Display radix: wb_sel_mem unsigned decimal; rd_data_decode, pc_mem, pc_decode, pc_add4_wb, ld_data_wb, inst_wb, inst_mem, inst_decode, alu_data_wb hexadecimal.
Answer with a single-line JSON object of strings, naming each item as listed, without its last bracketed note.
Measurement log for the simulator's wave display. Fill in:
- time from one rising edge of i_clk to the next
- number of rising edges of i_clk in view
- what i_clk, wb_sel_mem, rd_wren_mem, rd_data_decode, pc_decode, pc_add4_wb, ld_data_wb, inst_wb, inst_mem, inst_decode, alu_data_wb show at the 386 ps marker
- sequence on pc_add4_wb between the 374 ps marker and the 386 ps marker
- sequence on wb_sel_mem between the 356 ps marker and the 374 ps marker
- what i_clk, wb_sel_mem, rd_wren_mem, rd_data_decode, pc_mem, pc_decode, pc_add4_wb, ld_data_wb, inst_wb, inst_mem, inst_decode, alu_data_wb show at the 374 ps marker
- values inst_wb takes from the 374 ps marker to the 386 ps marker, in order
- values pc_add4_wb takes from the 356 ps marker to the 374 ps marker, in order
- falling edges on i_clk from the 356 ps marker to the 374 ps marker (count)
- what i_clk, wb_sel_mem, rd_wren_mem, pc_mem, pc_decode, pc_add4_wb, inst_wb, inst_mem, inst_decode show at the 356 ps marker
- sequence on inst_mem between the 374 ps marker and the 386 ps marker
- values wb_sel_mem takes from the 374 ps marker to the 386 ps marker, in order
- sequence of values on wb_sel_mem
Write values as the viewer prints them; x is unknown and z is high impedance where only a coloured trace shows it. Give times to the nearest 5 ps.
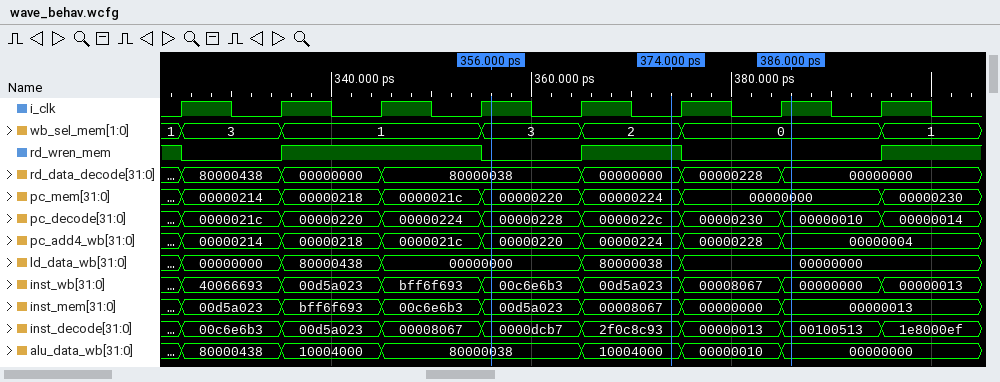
{"time from one rising edge of i_clk to the next": "10 ps", "number of rising edges of i_clk in view": "8", "what i_clk, wb_sel_mem, rd_wren_mem, rd_data_decode, pc_decode, pc_add4_wb, ld_data_wb, inst_wb, inst_mem, inst_decode, alu_data_wb show at the 386 ps marker": "i_clk=1, wb_sel_mem=0, rd_wren_mem=0, rd_data_decode=00000000, pc_decode=00000010, pc_add4_wb=00000004, ld_data_wb=00000000, inst_wb=00000000, inst_mem=00000013, inst_decode=00100513, alu_data_wb=00000000", "sequence on pc_add4_wb between the 374 ps marker and the 386 ps marker": "00000224, 00000228, 00000004", "sequence on wb_sel_mem between the 356 ps marker and the 374 ps marker": "3, 2", "what i_clk, wb_sel_mem, rd_wren_mem, rd_data_decode, pc_mem, pc_decode, pc_add4_wb, ld_data_wb, inst_wb, inst_mem, inst_decode, alu_data_wb show at the 374 ps marker": "i_clk=0, wb_sel_mem=2, rd_wren_mem=1, rd_data_decode=00000000, pc_mem=00000224, pc_decode=0000022c, pc_add4_wb=00000224, ld_data_wb=80000038, inst_wb=00d5a023, inst_mem=00008067, inst_decode=2f0c8c93, alu_data_wb=10004000", "values inst_wb takes from the 374 ps marker to the 386 ps marker, in order": "00d5a023, 00008067, 00000000", "values pc_add4_wb takes from the 356 ps marker to the 374 ps marker, in order": "00000220, 00000224", "falling edges on i_clk from the 356 ps marker to the 374 ps marker": "2", "what i_clk, wb_sel_mem, rd_wren_mem, pc_mem, pc_decode, pc_add4_wb, inst_wb, inst_mem, inst_decode show at the 356 ps marker": "i_clk=1, wb_sel_mem=3, rd_wren_mem=0, pc_mem=00000220, pc_decode=00000228, pc_add4_wb=00000220, inst_wb=00c6e6b3, inst_mem=00d5a023, inst_decode=0000dcb7", "sequence on inst_mem between the 374 ps marker and the 386 ps marker": "00008067, 00000000, 00000013", "values wb_sel_mem takes from the 374 ps marker to the 386 ps marker, in order": "2, 0", "sequence of values on wb_sel_mem": "1, 3, 1, 3, 2, 0, 1"}
